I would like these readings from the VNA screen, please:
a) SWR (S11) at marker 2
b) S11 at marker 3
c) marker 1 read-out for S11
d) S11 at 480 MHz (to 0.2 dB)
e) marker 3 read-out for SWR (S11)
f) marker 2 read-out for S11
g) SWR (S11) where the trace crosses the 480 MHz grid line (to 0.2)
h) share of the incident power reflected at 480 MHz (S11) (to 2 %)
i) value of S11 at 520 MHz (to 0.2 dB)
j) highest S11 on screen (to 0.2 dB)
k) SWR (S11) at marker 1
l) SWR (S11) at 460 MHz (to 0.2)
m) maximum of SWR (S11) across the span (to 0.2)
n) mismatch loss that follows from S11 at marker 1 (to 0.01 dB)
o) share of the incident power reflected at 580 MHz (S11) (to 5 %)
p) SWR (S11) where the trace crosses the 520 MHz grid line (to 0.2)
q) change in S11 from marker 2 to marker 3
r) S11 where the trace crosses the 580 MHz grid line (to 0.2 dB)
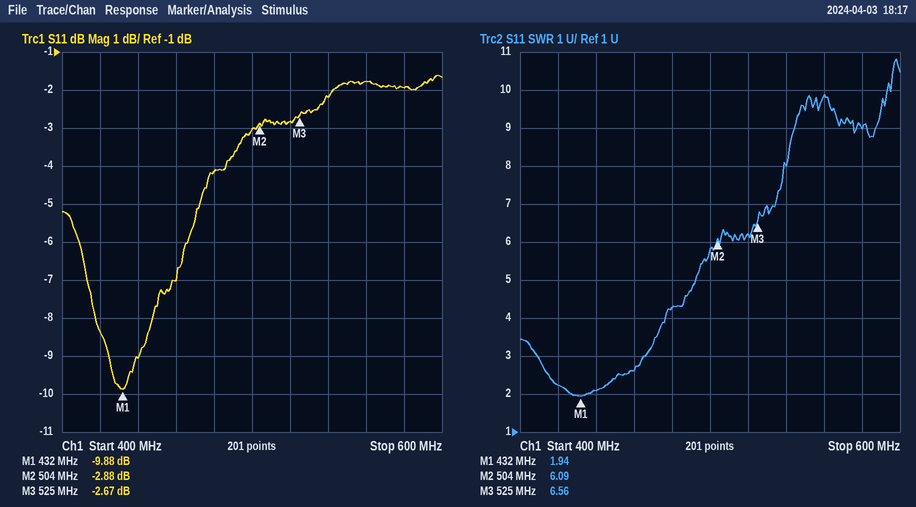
6.09
-2.67 dB
-9.88 dB
-4.2 dB
6.56
-2.88 dB
4.2
38 %
-2.8 dB
-1.6 dB
1.94
2.6
10.8
0.47 dB
65 %
6.2
0.21 dB
-2.0 dB
